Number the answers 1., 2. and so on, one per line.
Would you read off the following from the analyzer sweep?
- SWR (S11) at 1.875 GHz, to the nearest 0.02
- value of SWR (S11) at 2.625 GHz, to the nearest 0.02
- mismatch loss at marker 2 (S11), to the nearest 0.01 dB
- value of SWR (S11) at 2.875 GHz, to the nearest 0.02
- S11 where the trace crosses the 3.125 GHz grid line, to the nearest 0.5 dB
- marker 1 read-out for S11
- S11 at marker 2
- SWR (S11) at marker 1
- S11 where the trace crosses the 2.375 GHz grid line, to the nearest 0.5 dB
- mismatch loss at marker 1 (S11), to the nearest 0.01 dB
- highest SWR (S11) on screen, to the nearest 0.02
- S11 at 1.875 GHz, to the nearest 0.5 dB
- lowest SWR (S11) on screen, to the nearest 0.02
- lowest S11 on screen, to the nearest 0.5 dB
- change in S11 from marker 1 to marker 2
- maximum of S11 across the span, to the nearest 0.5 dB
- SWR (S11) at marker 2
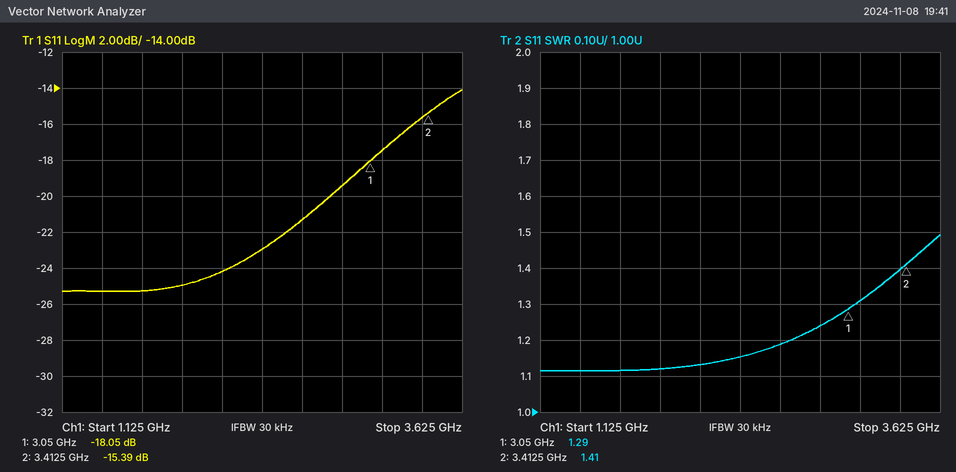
1. 1.12
2. 1.18
3. 0.13 dB
4. 1.24
5. -17.5 dB
6. -18.05 dB
7. -15.39 dB
8. 1.29
9. -23.0 dB
10. 0.07 dB
11. 1.50
12. -25.0 dB
13. 1.12
14. -25.5 dB
15. 2.66 dB
16. -14.0 dB
17. 1.41
